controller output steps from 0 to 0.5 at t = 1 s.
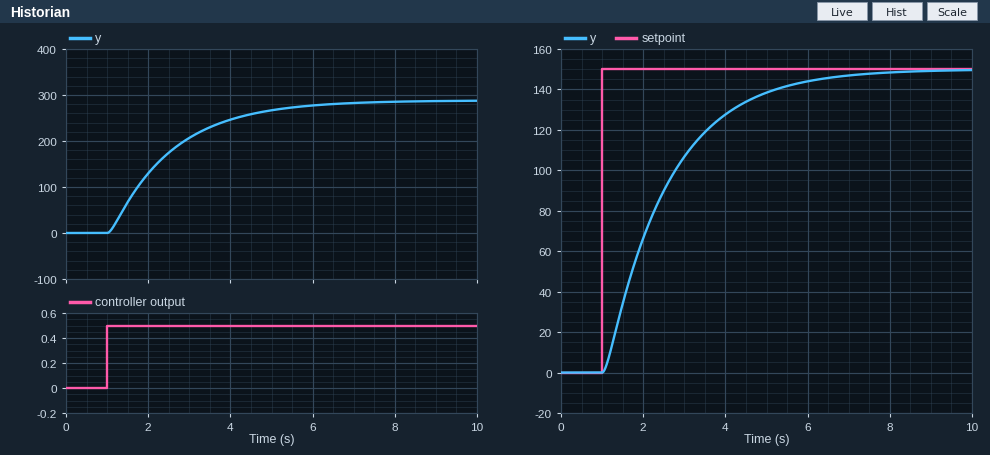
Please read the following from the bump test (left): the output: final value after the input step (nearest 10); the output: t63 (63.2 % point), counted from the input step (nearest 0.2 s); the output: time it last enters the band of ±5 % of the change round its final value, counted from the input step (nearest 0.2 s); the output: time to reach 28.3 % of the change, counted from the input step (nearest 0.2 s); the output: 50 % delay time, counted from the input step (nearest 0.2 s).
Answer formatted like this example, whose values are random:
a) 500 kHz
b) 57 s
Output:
a) 290
b) 1.6 s
c) 4.6 s
d) 0.6 s
e) 1.2 s
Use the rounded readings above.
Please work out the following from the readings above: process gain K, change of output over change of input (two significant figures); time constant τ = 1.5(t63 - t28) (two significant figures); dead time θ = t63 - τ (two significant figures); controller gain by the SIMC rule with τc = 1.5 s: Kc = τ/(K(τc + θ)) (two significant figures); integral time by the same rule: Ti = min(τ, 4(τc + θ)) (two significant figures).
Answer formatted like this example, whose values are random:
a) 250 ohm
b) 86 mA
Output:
a) 580
b) 1.5 s
c) 0.10 s
d) 0.0016
e) 1.5 s
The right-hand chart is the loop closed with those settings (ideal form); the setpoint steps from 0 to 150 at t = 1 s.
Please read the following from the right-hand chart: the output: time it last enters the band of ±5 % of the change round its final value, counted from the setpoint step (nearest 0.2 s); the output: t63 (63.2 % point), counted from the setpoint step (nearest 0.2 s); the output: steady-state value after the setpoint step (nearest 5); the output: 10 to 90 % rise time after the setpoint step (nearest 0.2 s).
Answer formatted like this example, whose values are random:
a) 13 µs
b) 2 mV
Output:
a) 4.6 s
b) 1.6 s
c) 150
d) 3.4 s
